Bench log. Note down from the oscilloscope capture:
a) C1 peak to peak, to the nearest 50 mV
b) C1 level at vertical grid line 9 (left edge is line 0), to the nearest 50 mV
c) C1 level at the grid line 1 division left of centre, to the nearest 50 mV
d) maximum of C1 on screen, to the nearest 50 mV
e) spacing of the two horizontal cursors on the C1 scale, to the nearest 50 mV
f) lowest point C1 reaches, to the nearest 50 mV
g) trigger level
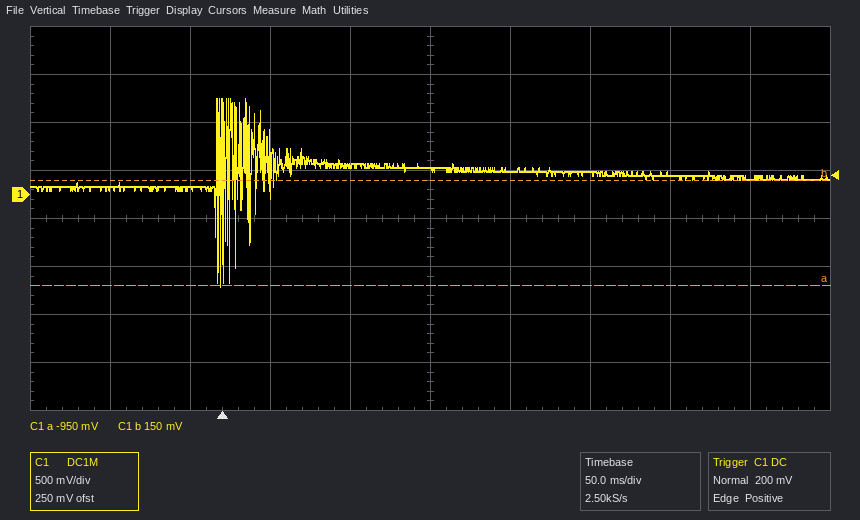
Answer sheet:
1.95 V
150 mV
300 mV
1.00 V
1.10 V
-950 mV
200 mV
